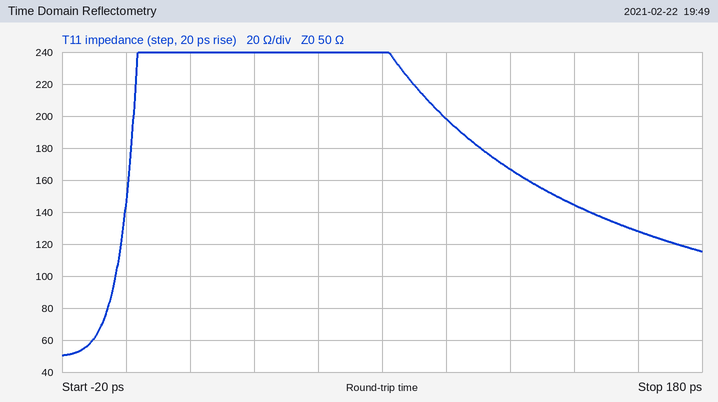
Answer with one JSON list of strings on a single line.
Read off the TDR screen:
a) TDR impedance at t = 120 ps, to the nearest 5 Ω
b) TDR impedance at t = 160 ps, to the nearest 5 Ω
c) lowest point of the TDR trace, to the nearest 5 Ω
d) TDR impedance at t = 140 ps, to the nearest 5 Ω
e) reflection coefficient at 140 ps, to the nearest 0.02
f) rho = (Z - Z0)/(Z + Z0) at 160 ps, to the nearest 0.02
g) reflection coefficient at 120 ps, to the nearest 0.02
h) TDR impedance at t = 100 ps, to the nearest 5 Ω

["165 Ω", "130 Ω", "50 Ω", "145 Ω", "+0.48", "+0.44", "+0.54", "200 Ω"]
